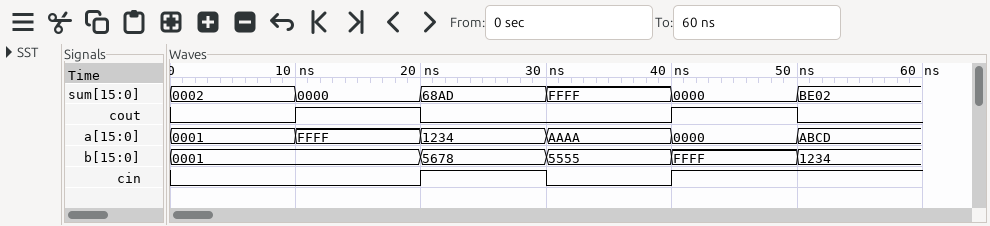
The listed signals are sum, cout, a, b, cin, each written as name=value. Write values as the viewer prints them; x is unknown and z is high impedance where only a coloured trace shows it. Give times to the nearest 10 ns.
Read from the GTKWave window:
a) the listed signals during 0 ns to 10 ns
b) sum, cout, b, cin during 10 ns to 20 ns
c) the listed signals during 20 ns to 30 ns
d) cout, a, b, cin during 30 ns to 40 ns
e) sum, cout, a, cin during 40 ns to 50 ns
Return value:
sum=0002, cout=0, a=0001, b=0001, cin=0
sum=0000, cout=1, b=0001, cin=0
sum=68AD, cout=0, a=1234, b=5678, cin=1
cout=0, a=AAAA, b=5555, cin=0
sum=0000, cout=1, a=0000, cin=1
